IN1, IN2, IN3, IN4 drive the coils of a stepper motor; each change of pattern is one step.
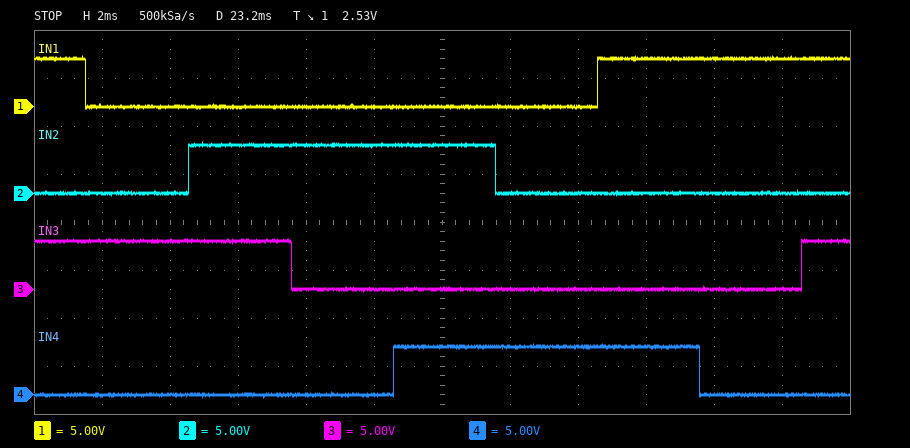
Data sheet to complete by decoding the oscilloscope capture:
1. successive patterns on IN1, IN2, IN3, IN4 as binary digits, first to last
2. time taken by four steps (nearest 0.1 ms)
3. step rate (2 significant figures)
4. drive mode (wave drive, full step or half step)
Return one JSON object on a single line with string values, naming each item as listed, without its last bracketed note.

{"successive patterns on IN1, IN2, IN3, IN4 as binary digits, first to last": "1010 0010 0110 0100 0101 0001 1001 1000 1010", "time taken by four steps": "12.1 ms", "step rate": "330 steps/s", "drive mode": "half step"}
